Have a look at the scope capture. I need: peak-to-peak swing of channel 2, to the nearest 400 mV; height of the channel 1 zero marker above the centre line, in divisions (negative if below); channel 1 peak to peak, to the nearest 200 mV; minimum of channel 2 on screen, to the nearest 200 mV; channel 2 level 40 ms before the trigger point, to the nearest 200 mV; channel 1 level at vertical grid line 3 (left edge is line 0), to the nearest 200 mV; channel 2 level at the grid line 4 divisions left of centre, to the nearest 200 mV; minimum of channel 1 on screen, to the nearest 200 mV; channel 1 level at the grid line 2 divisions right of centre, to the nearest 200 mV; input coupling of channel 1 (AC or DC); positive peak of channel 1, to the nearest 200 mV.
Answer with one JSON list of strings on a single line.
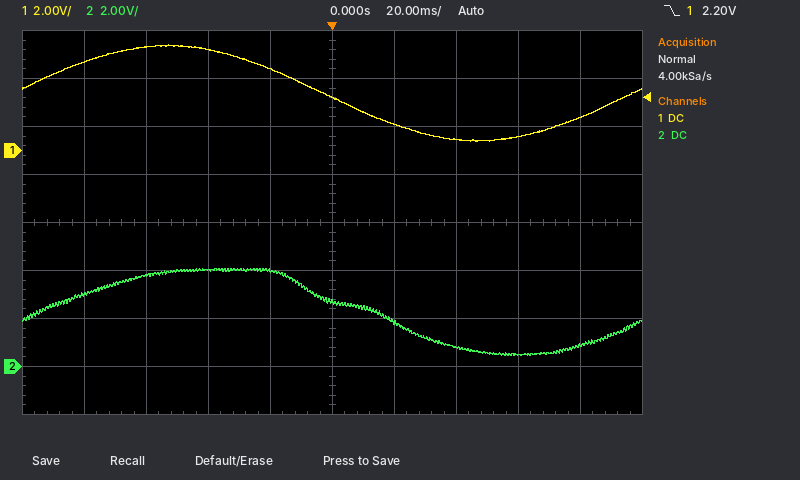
["3.6 V", "+1.5 div", "4.0 V", "400 mV", "4.0 V", "4.2 V", "3.0 V", "400 mV", "400 mV", "DC", "4.4 V"]
